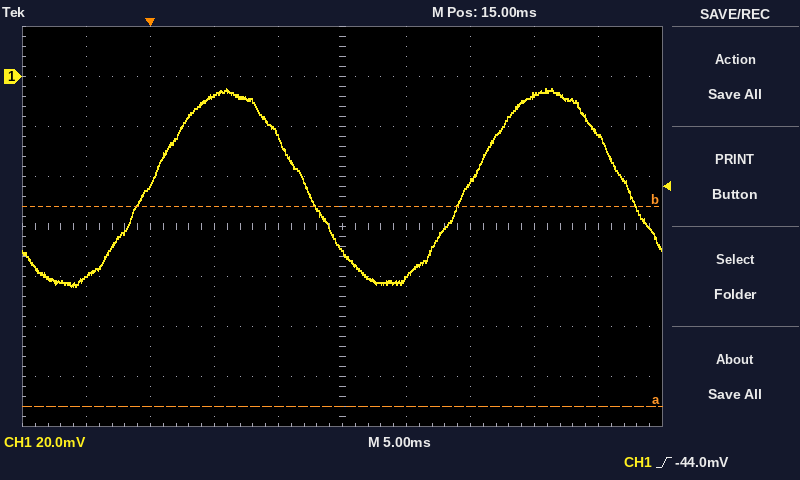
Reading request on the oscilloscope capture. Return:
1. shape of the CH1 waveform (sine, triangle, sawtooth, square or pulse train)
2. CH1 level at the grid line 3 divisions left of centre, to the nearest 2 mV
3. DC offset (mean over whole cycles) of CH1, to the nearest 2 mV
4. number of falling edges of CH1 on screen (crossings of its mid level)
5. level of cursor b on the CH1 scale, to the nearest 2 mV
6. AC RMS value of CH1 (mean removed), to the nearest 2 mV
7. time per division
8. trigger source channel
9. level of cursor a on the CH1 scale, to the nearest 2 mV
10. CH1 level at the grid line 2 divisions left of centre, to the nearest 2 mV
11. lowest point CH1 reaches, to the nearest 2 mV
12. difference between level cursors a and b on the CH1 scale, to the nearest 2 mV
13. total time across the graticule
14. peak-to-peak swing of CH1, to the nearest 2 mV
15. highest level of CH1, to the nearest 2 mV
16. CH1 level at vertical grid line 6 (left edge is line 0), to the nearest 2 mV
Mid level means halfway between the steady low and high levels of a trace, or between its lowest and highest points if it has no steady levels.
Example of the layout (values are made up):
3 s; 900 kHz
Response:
sine; -44 mV; -44 mV; 2; -52 mV; 28 mV; 5 ms; CH1; -132 mV; -8 mV; -84 mV; 80 mV; 50 ms; 80 mV; -4 mV; -80 mV
